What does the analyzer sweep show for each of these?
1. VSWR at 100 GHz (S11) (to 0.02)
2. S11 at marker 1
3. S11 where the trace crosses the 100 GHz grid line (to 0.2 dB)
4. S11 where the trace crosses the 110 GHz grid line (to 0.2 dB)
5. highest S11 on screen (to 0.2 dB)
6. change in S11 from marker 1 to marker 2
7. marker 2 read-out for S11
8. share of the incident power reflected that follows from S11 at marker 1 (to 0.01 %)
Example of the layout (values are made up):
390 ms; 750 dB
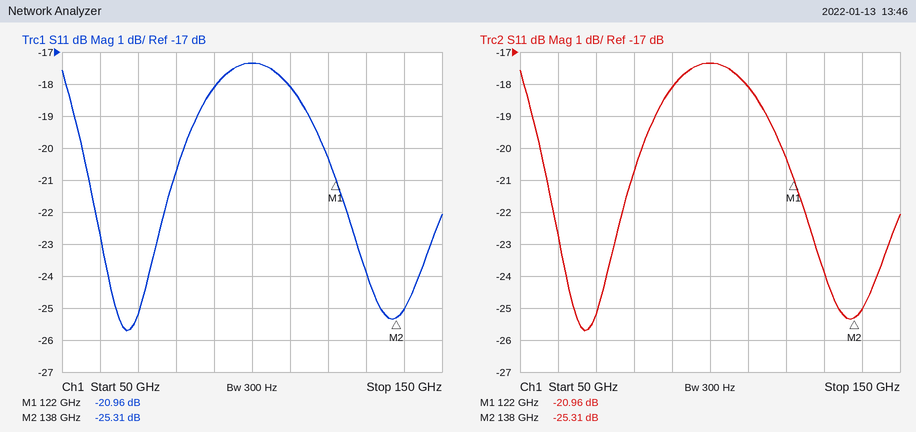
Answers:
1.32; -20.96 dB; -17.4 dB; -18.0 dB; -17.4 dB; -4.35 dB; -25.31 dB; 0.80 %
